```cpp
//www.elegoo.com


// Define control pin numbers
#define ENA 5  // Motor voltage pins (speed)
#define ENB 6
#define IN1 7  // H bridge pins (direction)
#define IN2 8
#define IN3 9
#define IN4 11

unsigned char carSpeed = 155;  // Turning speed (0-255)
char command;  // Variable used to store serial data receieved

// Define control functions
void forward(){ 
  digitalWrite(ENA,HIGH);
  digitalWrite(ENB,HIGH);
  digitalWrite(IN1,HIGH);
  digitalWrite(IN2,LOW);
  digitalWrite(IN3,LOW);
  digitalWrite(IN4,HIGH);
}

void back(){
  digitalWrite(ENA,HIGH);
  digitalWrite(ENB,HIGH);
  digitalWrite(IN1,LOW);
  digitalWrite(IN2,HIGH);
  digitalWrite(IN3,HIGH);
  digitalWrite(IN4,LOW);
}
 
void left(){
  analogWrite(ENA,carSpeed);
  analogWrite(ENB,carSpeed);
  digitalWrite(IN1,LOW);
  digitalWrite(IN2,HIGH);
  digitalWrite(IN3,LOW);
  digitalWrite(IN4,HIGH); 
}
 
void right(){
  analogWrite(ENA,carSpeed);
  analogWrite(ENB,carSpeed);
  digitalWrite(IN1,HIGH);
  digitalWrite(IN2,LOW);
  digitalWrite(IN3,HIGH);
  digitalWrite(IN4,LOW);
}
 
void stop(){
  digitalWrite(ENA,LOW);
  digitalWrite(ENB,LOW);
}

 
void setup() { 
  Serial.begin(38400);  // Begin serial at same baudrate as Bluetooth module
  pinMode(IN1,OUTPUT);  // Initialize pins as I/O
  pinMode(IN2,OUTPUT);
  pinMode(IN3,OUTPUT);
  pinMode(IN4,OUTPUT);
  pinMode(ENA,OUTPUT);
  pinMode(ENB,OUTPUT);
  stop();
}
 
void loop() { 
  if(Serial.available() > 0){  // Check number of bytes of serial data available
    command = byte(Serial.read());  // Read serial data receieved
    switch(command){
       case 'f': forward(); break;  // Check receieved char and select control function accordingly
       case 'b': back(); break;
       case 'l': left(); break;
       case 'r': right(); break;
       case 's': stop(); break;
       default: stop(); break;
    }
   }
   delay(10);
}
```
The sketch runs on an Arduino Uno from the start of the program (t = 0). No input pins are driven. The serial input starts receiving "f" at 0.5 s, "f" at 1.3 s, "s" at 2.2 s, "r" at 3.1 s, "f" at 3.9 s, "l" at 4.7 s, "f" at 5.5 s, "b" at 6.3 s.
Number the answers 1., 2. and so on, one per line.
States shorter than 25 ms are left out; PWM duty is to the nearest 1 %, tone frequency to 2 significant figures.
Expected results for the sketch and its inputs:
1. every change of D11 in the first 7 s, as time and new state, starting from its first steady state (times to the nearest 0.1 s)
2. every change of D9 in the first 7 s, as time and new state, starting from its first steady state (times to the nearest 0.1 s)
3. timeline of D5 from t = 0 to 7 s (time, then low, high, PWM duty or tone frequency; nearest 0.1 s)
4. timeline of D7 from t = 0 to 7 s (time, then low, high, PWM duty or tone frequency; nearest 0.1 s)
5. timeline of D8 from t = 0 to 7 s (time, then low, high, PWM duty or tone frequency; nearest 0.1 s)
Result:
1. 0 s low; 0.5 s high; 3.1 s low; 3.9 s high; 6.3 s low
2. 0 s low; 3.1 s high; 3.9 s low; 6.3 s high
3. 0 s low; 0.5 s high; 2.2 s low; 3.1 s PWM 61 %; 3.9 s high; 4.7 s PWM 61 %; 5.5 s high
4. 0 s low; 0.5 s high; 4.7 s low; 5.5 s high; 6.3 s low
5. 0 s low; 4.7 s high; 5.5 s low; 6.3 s high
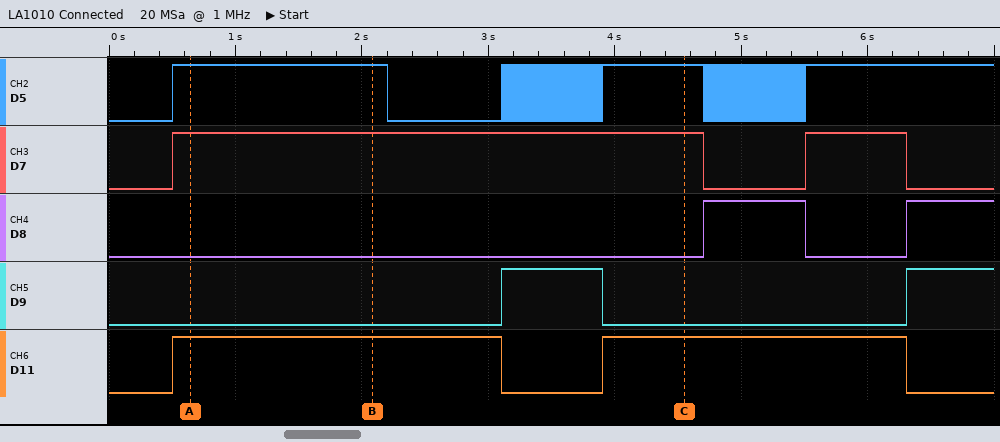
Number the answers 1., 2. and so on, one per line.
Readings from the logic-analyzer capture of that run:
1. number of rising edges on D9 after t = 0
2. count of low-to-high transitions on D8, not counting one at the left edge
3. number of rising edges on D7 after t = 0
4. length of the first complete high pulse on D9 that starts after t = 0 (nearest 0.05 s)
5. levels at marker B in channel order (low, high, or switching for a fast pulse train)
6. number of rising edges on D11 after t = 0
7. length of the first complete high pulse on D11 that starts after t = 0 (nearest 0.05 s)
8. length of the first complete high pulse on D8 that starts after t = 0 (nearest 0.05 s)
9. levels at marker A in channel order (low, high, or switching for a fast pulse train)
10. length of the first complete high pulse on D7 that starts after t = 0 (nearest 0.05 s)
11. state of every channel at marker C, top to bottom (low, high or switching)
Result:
1. 2
2. 2
3. 2
4. 0.80 s
5. D5 high, D7 high, D8 low, D9 low, D11 high
6. 2
7. 2.60 s
8. 0.80 s
9. D5 high, D7 high, D8 low, D9 low, D11 high
10. 4.20 s
11. D5 high, D7 high, D8 low, D9 low, D11 high
